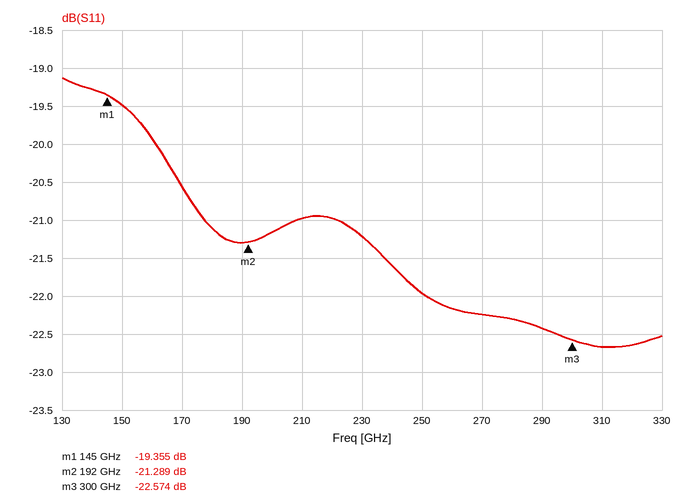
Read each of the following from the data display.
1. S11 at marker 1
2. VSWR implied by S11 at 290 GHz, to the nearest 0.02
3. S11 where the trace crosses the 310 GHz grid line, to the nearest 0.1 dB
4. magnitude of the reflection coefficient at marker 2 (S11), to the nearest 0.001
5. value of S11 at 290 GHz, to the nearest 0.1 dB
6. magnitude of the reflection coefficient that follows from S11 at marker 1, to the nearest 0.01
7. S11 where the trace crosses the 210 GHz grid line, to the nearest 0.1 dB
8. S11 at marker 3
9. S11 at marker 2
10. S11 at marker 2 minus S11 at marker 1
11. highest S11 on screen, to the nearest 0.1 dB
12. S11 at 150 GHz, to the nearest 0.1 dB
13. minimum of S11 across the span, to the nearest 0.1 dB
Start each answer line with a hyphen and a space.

- -19.355 dB
- 1.16
- -22.7 dB
- 0.086
- -22.4 dB
- 0.11
- -21.0 dB
- -22.574 dB
- -21.289 dB
- -1.934 dB
- -19.1 dB
- -19.5 dB
- -22.7 dB
